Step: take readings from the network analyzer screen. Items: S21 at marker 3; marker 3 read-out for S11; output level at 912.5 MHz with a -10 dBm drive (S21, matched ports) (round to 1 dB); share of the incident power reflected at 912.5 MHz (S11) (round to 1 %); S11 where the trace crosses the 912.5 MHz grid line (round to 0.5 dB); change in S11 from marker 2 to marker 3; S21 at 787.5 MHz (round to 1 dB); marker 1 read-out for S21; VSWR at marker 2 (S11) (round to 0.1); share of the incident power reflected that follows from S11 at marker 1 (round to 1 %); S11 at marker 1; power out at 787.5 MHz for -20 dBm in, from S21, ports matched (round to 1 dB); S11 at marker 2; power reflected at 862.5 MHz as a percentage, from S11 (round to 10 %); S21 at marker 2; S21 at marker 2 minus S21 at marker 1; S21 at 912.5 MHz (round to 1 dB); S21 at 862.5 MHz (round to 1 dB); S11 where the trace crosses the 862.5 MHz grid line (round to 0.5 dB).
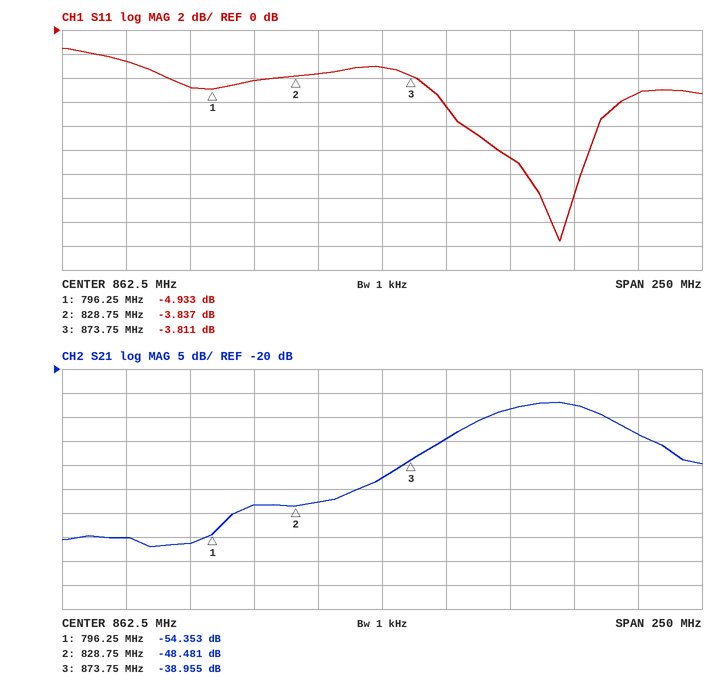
-38.955 dB
-3.811 dB
-38 dBm
9 %
-10.5 dB
0.026 dB
-56 dB
-54.353 dB
4.6
32 %
-4.933 dB
-76 dBm
-3.837 dB
50 %
-48.481 dB
5.872 dB
-28 dB
-43 dB
-3.0 dB
